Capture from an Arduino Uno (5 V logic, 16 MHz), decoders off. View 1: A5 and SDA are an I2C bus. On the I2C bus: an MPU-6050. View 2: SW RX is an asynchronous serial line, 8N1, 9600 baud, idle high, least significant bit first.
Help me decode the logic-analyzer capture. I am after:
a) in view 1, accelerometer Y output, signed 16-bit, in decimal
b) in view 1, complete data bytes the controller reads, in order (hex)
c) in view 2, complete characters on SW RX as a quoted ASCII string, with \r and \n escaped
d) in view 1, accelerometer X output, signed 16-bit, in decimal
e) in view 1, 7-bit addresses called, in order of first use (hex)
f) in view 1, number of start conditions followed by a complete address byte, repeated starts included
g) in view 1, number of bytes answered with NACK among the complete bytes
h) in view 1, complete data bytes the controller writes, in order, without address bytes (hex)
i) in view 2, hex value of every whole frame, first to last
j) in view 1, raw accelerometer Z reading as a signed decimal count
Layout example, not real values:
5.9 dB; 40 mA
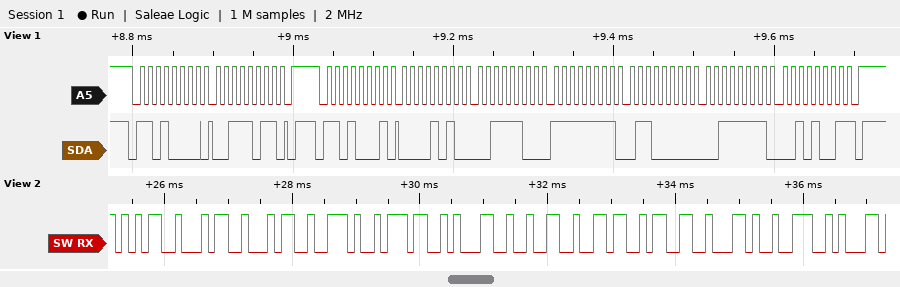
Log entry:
-160; 0A 3C FF 60 3F 29; "544.71263,N"; 2620; 0x68; 2; 1; 3B; 35 34 34 2E 37 31 32 36 33 2C 4E; 16169
